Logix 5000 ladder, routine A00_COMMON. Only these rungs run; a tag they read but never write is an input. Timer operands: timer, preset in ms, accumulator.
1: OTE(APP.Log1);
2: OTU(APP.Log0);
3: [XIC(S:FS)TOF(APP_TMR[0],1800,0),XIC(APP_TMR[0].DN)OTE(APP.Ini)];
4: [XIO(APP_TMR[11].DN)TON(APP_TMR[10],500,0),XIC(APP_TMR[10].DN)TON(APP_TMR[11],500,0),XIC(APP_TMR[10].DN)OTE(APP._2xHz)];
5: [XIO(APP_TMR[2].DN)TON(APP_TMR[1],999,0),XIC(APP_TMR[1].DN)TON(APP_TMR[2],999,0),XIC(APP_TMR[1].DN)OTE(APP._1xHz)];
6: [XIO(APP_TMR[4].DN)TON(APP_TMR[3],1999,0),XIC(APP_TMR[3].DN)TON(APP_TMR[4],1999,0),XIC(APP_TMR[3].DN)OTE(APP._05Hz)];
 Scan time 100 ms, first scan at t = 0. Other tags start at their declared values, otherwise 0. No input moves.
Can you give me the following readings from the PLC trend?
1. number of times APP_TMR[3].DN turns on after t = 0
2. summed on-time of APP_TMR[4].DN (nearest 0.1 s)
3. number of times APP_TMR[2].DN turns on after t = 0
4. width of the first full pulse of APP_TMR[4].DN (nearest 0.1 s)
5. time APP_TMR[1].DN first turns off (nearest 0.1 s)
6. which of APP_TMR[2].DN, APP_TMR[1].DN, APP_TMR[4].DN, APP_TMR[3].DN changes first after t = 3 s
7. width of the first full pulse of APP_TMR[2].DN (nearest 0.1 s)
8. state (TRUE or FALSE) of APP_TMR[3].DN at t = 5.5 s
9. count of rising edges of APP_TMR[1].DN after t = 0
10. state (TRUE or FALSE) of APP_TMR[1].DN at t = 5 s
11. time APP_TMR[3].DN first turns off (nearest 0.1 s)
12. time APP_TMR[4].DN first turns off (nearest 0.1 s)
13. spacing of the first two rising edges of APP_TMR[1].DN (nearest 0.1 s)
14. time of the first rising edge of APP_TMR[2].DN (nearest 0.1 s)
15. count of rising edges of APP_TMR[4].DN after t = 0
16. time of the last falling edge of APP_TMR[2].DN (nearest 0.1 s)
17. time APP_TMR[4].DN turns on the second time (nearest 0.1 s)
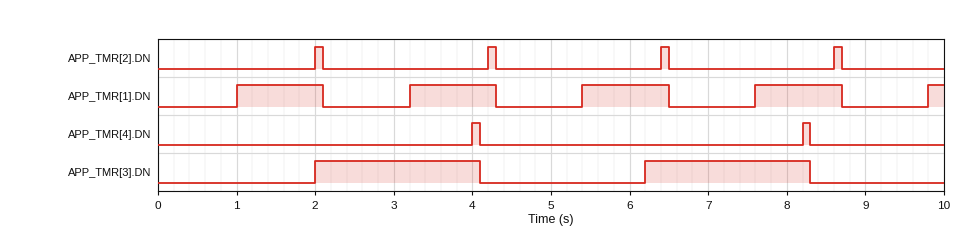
2
0.2 s
4
0.1 s
2.1 s
APP_TMR[1].DN
0.1 s
FALSE
5
FALSE
4.1 s
4.1 s
2.2 s
2.0 s
2
8.7 s
8.2 s
